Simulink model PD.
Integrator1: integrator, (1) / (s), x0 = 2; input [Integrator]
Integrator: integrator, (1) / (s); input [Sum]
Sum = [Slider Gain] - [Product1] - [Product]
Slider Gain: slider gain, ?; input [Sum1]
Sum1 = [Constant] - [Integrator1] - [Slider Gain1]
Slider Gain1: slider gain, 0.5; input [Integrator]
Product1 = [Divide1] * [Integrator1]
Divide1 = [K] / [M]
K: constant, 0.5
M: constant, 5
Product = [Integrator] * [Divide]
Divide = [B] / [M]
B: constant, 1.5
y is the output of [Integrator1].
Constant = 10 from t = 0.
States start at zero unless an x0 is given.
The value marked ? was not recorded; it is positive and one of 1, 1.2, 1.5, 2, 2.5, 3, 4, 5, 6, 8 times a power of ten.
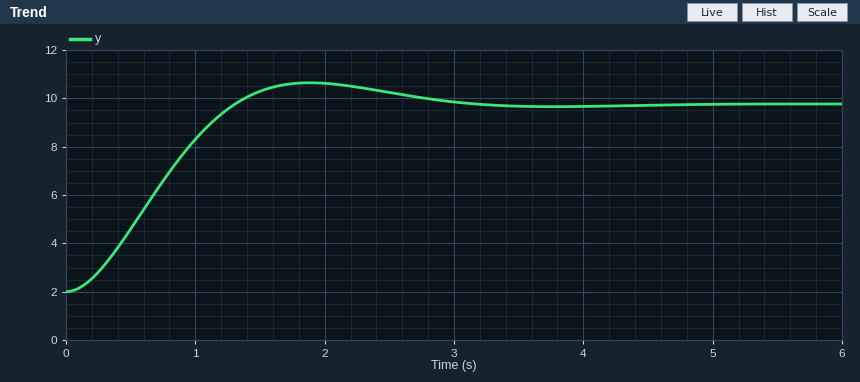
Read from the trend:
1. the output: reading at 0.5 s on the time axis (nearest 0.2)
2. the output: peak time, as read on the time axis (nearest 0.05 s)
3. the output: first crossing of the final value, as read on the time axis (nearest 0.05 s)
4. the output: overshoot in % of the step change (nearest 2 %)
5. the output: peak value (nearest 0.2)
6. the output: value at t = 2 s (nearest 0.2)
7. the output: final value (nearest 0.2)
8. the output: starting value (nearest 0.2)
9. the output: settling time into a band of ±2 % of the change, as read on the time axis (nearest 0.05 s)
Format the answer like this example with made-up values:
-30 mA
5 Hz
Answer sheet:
4.6
1.90 s
1.30 s
12 %
10.6
10.6
9.8
2.0
2.90 s
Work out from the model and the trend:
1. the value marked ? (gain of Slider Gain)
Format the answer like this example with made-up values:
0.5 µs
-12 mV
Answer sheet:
4
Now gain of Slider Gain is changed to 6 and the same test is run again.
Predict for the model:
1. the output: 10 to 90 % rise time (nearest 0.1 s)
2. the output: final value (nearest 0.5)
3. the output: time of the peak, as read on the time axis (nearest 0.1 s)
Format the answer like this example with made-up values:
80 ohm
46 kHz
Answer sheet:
0.8 s
10.0
1.7 s
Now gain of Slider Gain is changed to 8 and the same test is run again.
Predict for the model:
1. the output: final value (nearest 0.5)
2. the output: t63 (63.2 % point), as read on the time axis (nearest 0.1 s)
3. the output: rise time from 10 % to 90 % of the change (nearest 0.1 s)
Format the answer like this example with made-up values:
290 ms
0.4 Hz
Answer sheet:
10.0
0.6 s
0.8 s
